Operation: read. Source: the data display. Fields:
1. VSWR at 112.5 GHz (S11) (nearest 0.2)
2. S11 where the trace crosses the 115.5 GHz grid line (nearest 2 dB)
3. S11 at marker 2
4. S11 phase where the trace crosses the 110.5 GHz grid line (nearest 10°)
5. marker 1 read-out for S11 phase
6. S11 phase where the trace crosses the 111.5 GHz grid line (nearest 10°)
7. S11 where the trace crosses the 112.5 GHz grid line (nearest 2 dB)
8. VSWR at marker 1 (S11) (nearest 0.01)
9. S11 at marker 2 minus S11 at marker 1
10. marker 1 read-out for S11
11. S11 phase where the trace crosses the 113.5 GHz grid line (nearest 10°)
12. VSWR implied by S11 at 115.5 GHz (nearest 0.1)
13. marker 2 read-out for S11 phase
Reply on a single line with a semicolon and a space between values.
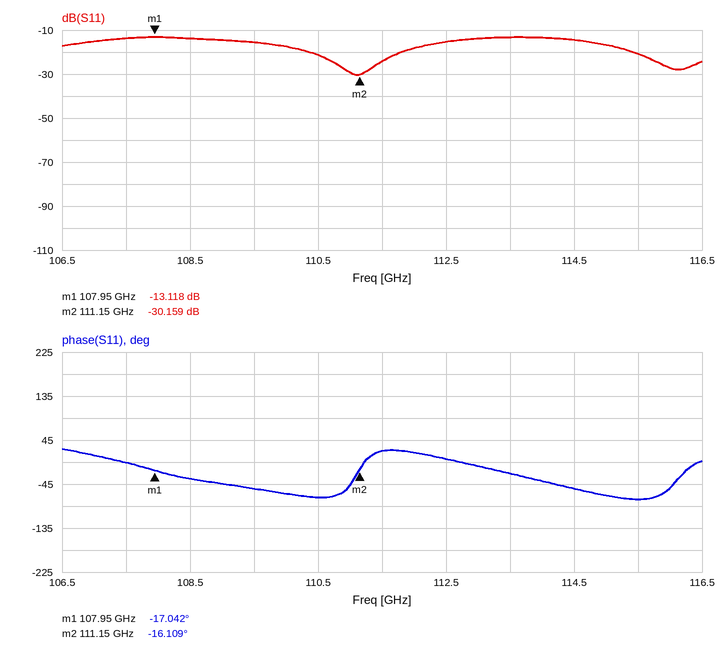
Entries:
1.4; -20 dB; -30.159 dB; -70°; -17.042°; 20°; -16 dB; 1.57; -17.041 dB; -13.118 dB; -20°; 1.2; -16.109°
